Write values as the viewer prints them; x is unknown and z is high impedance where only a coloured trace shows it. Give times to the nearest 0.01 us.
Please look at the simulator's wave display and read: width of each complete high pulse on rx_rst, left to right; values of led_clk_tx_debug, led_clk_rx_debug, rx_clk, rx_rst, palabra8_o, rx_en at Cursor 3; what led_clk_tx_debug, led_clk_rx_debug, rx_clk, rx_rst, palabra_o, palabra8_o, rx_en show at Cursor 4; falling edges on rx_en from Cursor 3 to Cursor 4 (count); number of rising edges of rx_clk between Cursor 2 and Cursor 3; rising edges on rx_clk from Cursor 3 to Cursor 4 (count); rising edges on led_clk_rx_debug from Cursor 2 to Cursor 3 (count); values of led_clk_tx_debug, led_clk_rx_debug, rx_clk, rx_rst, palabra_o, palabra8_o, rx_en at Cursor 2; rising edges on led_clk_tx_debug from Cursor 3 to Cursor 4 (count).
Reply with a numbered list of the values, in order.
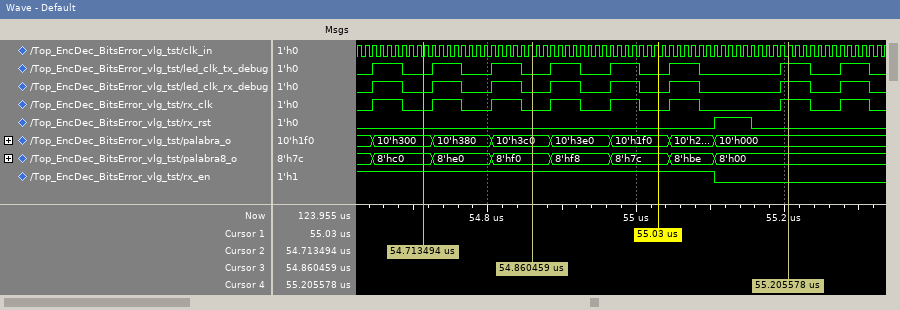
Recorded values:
1. 0.05 us
2. led_clk_tx_debug=0, led_clk_rx_debug=0, rx_clk=0, rx_rst=0, palabra8_o=8'hf0, rx_en=1
3. led_clk_tx_debug=1, led_clk_rx_debug=1, rx_clk=1, rx_rst=0, palabra_o=10'h000, palabra8_o=8'h00, rx_en=0
4. 1
5. 2
6. 4
7. 2
8. led_clk_tx_debug=0, led_clk_rx_debug=0, rx_clk=0, rx_rst=0, palabra_o=10'h300, palabra8_o=8'hc0, rx_en=1
9. 4
